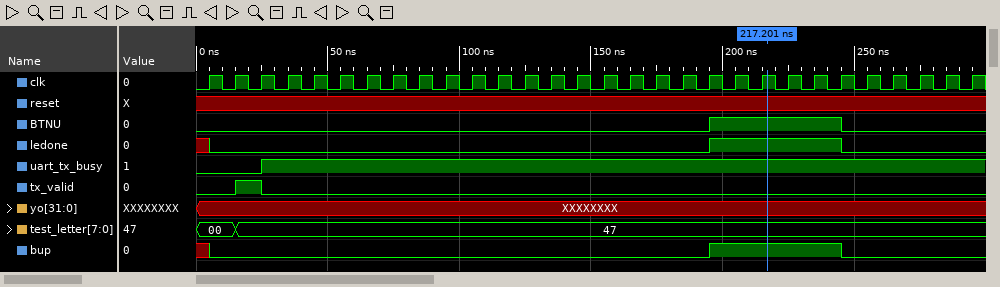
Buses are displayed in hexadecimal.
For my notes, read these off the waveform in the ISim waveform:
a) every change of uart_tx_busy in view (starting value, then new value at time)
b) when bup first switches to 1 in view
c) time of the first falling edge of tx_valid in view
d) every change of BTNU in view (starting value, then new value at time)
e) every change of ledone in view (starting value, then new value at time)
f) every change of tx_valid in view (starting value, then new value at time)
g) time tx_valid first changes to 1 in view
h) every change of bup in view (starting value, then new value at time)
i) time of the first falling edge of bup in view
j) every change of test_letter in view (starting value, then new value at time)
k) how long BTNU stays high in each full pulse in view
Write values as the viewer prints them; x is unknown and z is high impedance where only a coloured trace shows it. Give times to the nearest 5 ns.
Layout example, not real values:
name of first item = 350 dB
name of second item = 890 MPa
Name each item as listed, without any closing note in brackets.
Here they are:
every change of uart_tx_busy in view = 0, 1 at 25 ns
when bup first switches to 1 in view = 195 ns
time of the first falling edge of tx_valid in view = 25 ns
every change of BTNU in view = 0, 1 at 195 ns, 0 at 245 ns
every change of ledone in view = x, 0 at 5 ns, 1 at 195 ns, 0 at 245 ns
every change of tx_valid in view = 0, 1 at 15 ns, 0 at 25 ns
time tx_valid first changes to 1 in view = 15 ns
every change of bup in view = x, 0 at 5 ns, 1 at 195 ns, 0 at 245 ns
time of the first falling edge of bup in view = 245 ns
every change of test_letter in view = 00, 47 at 15 ns
how long BTNU stays high in each full pulse in view = 50 ns
